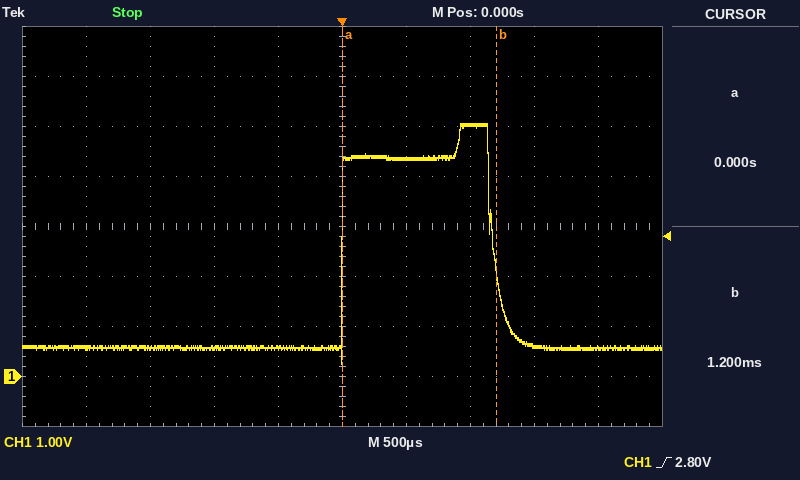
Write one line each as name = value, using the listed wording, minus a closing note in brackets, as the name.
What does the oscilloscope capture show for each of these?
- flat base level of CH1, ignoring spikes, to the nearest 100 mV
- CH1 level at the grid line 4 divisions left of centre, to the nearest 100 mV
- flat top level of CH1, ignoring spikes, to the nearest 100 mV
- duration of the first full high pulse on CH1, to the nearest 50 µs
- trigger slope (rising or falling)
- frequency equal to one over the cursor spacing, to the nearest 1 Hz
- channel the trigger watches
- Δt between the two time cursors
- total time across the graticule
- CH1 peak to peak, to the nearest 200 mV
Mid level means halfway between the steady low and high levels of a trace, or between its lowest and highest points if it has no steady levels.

flat base level of CH1, ignoring spikes, to the nearest 100 mV = 600 mV
CH1 level at the grid line 4 divisions left of centre, to the nearest 100 mV = 600 mV
flat top level of CH1, ignoring spikes, to the nearest 100 mV = 4.4 V
duration of the first full high pulse on CH1, to the nearest 50 µs = 1.20 ms
trigger slope = rising
frequency equal to one over the cursor spacing, to the nearest 1 Hz = 833 Hz
channel the trigger watches = CH1
Δt between the two time cursors = 1.20 ms
total time across the graticule = 5 ms
CH1 peak to peak, to the nearest 200 mV = 4.8 V
